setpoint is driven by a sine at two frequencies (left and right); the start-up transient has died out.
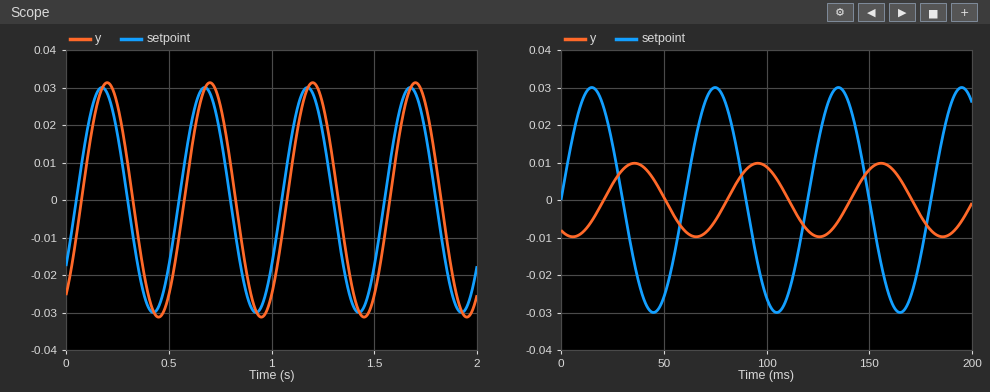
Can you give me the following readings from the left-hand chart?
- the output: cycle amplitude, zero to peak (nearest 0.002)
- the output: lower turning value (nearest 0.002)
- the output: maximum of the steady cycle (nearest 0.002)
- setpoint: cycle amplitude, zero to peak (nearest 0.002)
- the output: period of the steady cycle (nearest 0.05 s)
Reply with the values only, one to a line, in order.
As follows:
0.032
-0.032
0.032
0.030
0.50 s
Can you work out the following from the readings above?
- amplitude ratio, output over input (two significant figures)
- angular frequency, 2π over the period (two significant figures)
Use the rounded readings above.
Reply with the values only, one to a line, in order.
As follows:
1.1
13 rad/s
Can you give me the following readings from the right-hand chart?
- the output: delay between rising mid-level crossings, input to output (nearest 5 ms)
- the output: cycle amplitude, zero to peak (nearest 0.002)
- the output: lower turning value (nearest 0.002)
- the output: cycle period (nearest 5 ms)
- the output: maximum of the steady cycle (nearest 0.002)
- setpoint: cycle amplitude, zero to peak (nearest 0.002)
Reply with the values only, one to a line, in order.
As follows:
20 ms
0.010
-0.010
60 ms
0.010
0.030
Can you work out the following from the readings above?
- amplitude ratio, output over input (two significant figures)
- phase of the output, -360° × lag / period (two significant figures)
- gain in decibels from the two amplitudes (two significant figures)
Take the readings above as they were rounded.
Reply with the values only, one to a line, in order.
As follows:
0.33
-120°
-9.5 dB
